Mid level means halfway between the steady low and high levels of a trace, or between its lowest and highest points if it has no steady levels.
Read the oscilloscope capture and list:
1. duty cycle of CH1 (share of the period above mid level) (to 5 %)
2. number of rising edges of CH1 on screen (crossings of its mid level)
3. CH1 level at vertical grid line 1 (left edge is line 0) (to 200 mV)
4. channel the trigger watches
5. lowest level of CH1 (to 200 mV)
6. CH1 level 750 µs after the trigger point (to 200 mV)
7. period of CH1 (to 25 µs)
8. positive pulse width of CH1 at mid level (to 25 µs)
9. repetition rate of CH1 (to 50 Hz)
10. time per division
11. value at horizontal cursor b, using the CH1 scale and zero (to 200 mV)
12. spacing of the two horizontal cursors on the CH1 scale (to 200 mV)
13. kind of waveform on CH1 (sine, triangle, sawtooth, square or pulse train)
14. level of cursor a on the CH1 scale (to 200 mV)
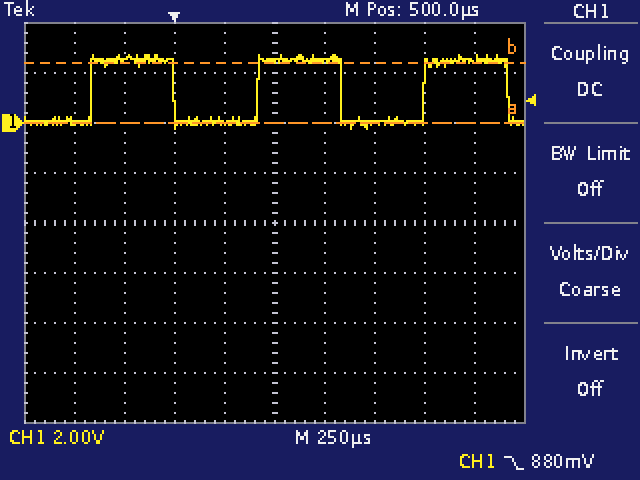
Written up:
50 %
3
0.0 V
CH1
-200 mV
2.4 V
825 µs
425 µs
1.20 kHz
250 µs
2.4 V
2.4 V
square
0.0 V
